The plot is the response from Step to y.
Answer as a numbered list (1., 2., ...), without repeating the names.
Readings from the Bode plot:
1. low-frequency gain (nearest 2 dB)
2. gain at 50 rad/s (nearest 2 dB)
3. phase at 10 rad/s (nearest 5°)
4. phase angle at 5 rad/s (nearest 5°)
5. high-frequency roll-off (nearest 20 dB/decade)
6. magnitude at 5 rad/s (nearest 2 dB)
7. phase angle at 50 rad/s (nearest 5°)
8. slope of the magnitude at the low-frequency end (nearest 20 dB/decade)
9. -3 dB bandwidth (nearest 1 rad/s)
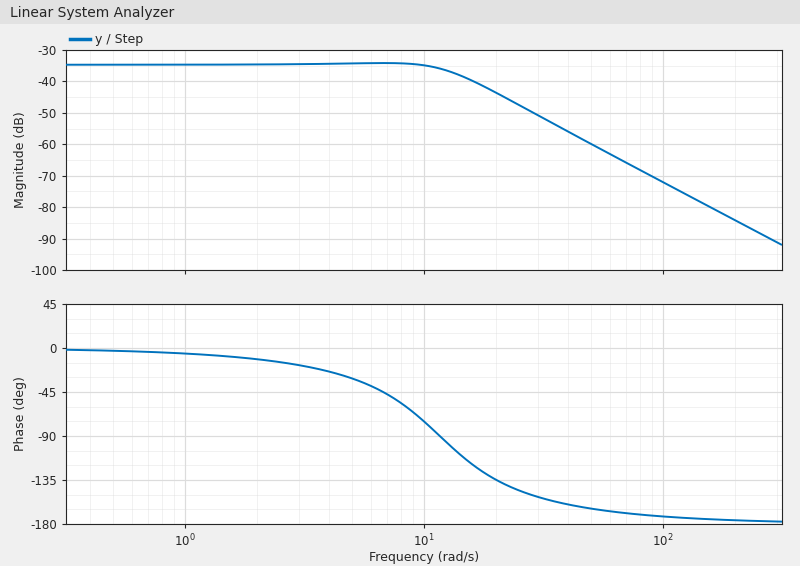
1. -34 dB
2. -60 dB
3. -75°
4. -30°
5. -40 dB/decade
6. -34 dB
7. -165°
8. 0 dB/decade
9. 14 rad/s
